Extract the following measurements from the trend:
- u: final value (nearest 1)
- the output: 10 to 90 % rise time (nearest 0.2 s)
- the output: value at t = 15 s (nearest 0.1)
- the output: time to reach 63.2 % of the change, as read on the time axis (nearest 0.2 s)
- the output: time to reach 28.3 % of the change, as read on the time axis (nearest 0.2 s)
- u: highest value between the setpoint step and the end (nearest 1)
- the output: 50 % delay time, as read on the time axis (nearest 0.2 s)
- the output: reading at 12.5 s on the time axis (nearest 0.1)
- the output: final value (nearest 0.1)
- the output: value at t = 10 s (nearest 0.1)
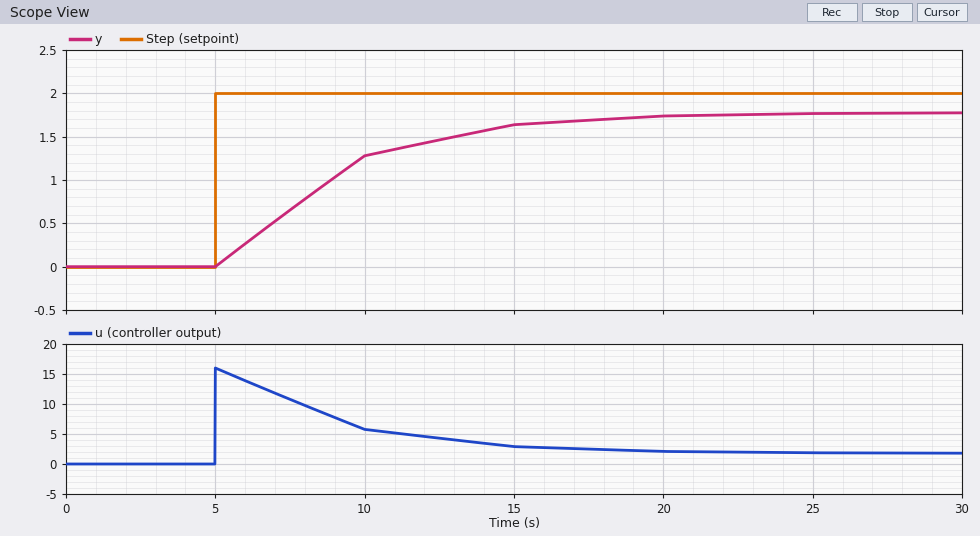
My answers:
2
8.8 s
1.6
9.4 s
7.0 s
16
8.4 s
1.5
1.8
1.3
